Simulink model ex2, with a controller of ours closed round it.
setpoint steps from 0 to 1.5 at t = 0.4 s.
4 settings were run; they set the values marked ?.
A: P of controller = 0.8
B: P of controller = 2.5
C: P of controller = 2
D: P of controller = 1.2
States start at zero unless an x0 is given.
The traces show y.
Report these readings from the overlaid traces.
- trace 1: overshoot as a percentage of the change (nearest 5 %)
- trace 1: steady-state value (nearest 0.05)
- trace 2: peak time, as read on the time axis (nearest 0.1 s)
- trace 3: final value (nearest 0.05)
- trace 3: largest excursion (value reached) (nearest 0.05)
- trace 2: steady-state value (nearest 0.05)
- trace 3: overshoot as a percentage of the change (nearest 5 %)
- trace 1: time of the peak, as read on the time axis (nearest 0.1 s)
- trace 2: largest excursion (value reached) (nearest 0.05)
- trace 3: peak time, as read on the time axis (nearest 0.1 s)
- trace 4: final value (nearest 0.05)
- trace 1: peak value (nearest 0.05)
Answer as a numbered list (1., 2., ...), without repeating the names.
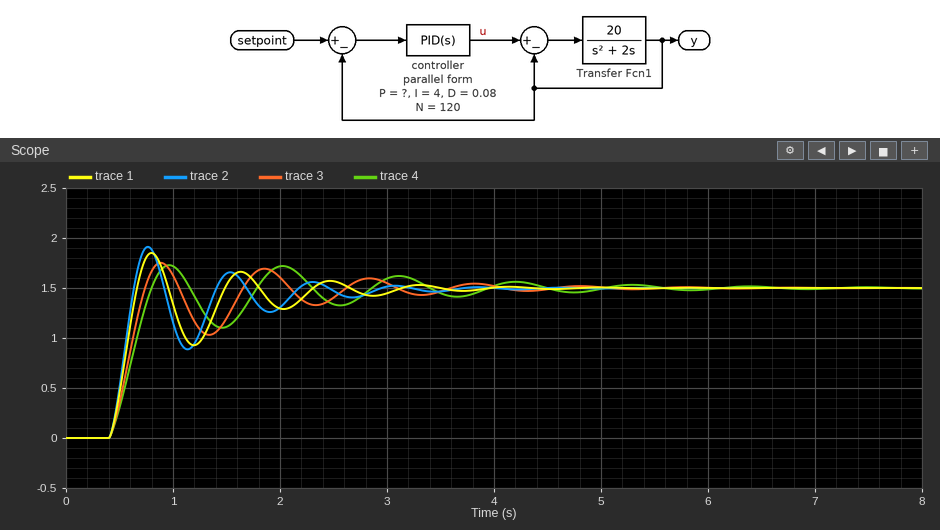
1. 25 %
2. 1.50
3. 0.8 s
4. 1.50
5. 1.75
6. 1.50
7. 15 %
8. 0.8 s
9. 1.90
10. 0.9 s
11. 1.50
12. 1.85
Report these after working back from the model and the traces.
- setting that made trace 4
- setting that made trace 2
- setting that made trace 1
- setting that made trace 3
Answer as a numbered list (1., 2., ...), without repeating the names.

1. A
2. B
3. C
4. D
